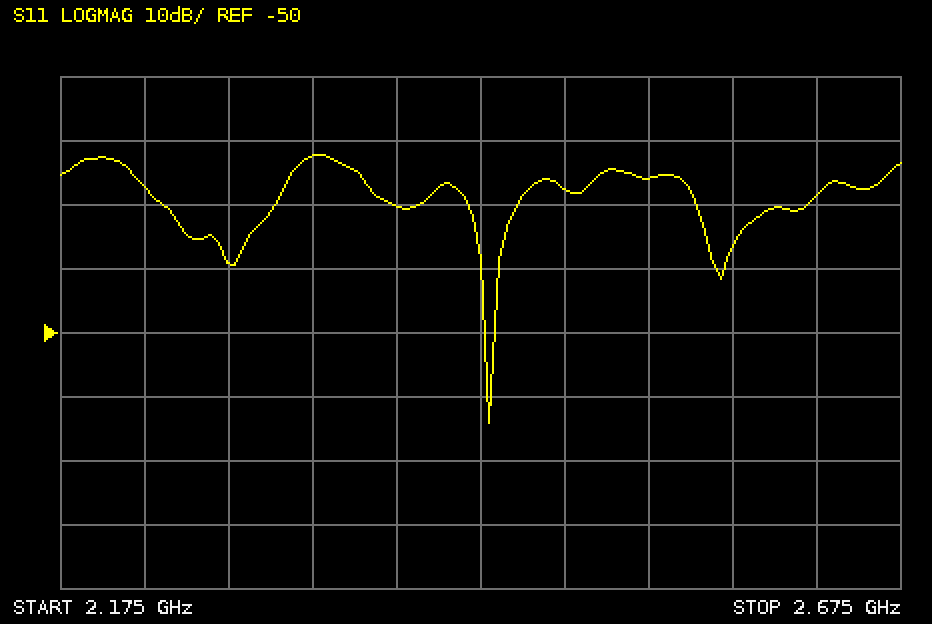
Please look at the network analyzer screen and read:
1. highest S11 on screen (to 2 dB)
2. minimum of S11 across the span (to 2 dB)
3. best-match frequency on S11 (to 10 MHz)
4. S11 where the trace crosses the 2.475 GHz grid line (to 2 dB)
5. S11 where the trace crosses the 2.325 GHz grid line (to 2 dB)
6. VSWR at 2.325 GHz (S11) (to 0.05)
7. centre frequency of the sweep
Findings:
-22 dB
-64 dB
2.43 GHz
-28 dB
-22 dB
1.15
2.425 GHz
